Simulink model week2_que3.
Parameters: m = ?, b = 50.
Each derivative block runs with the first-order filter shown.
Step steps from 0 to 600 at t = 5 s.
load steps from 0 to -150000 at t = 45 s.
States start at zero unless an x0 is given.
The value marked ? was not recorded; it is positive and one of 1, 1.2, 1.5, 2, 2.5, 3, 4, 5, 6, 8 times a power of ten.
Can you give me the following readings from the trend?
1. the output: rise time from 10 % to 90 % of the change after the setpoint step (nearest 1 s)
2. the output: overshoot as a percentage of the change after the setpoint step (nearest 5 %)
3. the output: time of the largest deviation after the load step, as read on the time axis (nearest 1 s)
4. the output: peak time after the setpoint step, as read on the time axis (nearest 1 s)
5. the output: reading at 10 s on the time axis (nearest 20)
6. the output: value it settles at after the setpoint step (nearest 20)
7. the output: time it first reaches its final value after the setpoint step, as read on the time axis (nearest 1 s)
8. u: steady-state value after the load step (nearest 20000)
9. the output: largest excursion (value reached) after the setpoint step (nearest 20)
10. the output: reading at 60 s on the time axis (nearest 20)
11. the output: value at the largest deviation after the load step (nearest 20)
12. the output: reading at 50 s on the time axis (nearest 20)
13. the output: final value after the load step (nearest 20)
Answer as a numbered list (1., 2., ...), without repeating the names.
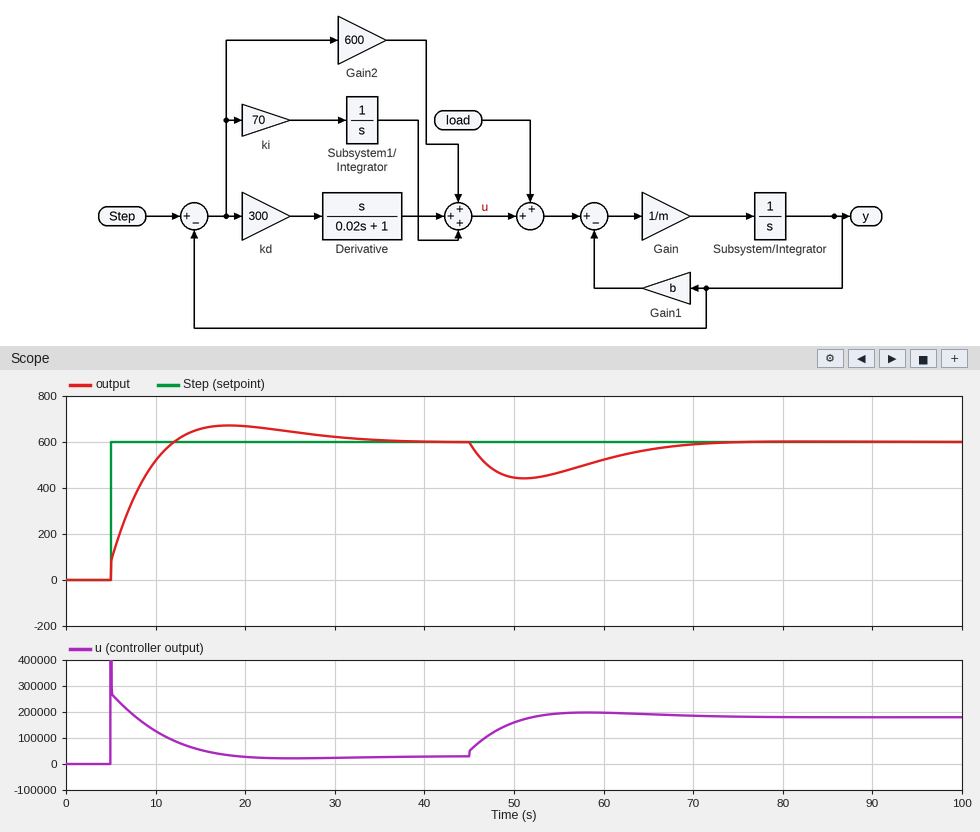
1. 5 s
2. 10 %
3. 51 s
4. 18 s
5. 520
6. 600
7. 12 s
8. 180000
9. 680
10. 520
11. 440
12. 440
13. 600
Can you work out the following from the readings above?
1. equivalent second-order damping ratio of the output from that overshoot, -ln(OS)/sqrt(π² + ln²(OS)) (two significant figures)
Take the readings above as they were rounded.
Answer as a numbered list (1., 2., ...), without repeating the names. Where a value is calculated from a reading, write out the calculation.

1. ln(0.1) = -2.303; 2.303 / sqrt(9.870 + 5.302) = 0.59
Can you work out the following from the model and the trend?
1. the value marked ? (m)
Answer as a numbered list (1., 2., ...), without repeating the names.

1. 2000
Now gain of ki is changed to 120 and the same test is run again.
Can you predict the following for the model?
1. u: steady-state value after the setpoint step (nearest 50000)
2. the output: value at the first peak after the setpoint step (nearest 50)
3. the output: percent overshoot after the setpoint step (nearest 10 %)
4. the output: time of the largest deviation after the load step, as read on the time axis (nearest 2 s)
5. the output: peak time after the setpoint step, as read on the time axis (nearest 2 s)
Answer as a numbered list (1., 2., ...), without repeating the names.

1. 50000
2. 700
3. 20 %
4. 50 s
5. 16 s
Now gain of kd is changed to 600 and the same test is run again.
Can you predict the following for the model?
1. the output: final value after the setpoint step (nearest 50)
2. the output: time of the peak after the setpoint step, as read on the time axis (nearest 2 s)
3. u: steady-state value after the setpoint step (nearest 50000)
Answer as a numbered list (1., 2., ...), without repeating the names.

1. 600
2. 20 s
3. 50000
